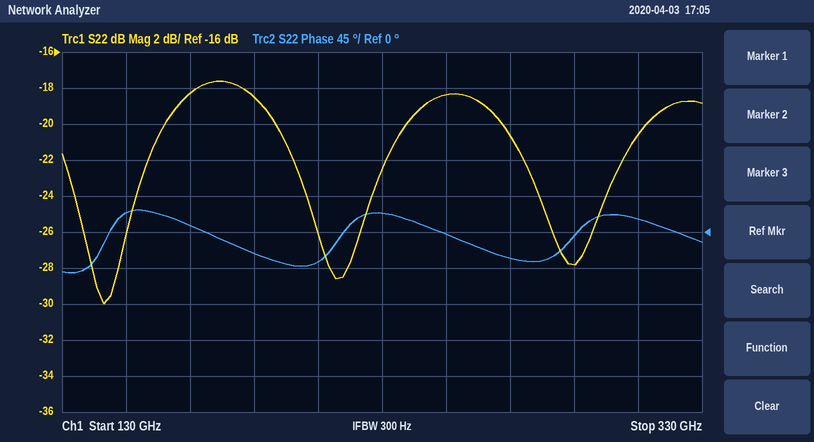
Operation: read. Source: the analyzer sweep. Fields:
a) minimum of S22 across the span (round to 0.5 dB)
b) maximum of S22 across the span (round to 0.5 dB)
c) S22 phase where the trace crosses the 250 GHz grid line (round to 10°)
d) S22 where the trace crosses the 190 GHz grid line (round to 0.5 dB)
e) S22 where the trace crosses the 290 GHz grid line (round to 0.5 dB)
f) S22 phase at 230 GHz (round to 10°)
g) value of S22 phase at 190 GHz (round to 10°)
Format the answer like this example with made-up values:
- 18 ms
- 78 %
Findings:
- -30.0 dB
- -17.5 dB
- 0°
- -18.5 dB
- -28.0 dB
- 20°
- -30°
